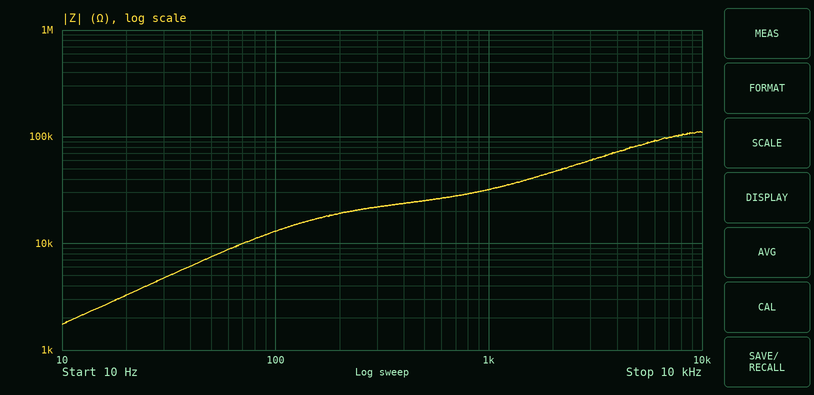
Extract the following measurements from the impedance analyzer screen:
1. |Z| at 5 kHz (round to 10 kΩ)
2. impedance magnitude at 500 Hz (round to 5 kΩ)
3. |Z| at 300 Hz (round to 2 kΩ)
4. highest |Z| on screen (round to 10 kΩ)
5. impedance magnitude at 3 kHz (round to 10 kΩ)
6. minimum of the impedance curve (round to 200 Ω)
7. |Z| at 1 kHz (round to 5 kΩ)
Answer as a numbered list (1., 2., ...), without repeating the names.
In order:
1. 80 kΩ
2. 25 kΩ
3. 22 kΩ
4. 110 kΩ
5. 60 kΩ
6. 1.8 kΩ
7. 30 kΩ
